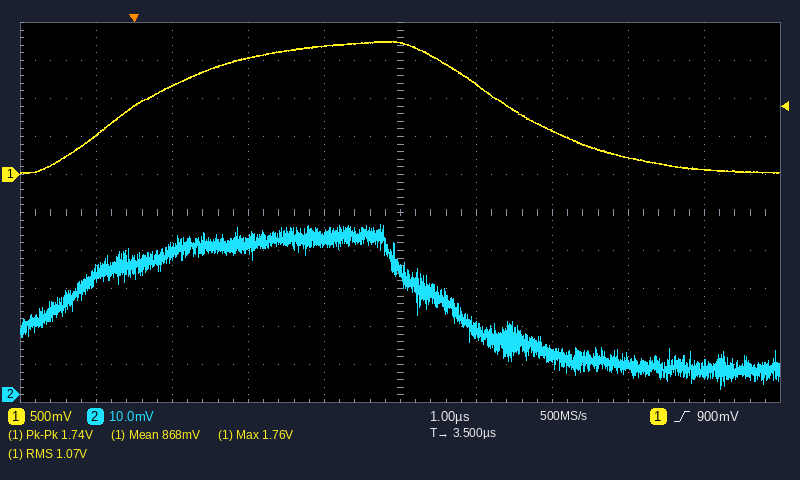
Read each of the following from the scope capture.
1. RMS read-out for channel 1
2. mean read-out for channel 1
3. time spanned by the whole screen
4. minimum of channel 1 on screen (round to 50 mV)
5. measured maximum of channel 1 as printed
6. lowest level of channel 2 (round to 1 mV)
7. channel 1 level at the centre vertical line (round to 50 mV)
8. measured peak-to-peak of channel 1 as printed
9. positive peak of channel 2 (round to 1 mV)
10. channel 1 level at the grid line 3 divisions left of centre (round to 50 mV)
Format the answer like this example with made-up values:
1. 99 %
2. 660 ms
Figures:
1. 1.07 V
2. 868 mV
3. 10 µs
4. 0 mV
5. 1.76 V
6. 1 mV
7. 1.75 V
8. 1.74 V
9. 45 mV
10. 1.15 V
